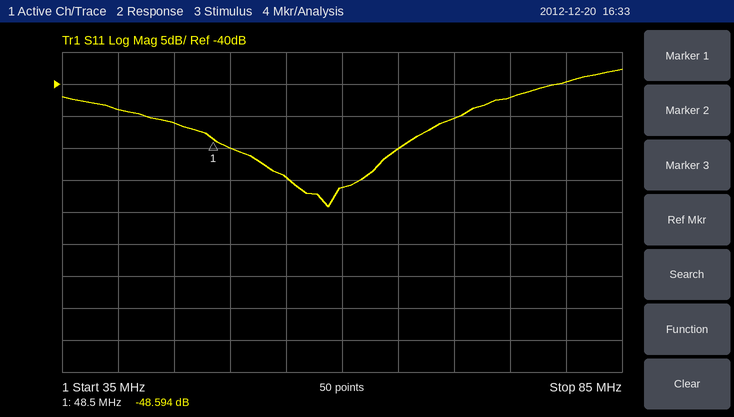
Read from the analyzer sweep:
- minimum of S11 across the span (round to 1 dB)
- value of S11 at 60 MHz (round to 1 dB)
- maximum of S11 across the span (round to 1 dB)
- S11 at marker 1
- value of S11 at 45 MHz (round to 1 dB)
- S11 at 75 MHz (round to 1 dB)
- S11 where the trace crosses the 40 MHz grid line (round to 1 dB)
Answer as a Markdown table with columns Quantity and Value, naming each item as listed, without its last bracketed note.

| Quantity | Value |
|---|---|
| minimum of S11 across the span | -59 dB |
| value of S11 at 60 MHz | -56 dB |
| maximum of S11 across the span | -38 dB |
| S11 at marker 1 | -48.594 dB |
| value of S11 at 45 MHz | -46 dB |
| S11 at 75 MHz | -42 dB |
| S11 where the trace crosses the 40 MHz grid line | -44 dB |
